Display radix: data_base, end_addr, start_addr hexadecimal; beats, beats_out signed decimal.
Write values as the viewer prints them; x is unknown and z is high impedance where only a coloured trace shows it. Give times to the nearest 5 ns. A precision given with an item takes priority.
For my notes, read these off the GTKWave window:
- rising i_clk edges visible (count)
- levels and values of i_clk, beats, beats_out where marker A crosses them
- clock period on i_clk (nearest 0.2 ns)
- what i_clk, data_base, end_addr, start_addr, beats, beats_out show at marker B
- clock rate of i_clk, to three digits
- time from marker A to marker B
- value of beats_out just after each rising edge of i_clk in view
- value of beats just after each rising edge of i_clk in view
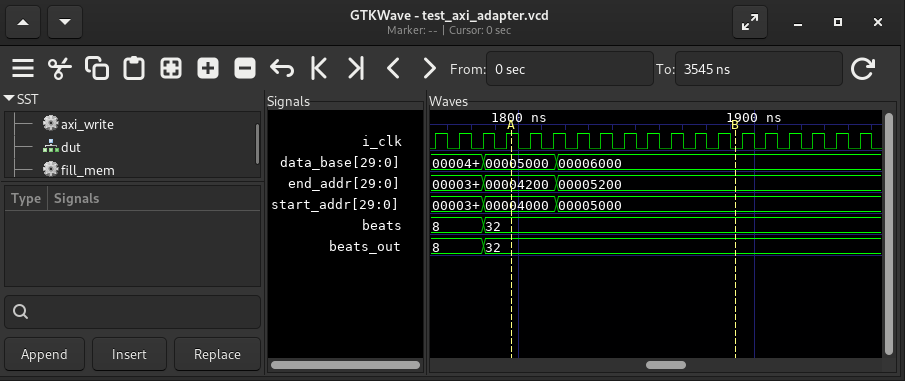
19
i_clk=1, beats=32, beats_out=32
10 ns
i_clk=0, data_base=00006000, end_addr=00005200, start_addr=00005000, beats=32, beats_out=32
100 MHz
95 ns
8, 8, 32, 32, 32, 32, 32, 32, 32, 32, 32, 32, 32, 32, 32, 32, 32, 32, 32
8, 8, 32, 32, 32, 32, 32, 32, 32, 32, 32, 32, 32, 32, 32, 32, 32, 32, 32
